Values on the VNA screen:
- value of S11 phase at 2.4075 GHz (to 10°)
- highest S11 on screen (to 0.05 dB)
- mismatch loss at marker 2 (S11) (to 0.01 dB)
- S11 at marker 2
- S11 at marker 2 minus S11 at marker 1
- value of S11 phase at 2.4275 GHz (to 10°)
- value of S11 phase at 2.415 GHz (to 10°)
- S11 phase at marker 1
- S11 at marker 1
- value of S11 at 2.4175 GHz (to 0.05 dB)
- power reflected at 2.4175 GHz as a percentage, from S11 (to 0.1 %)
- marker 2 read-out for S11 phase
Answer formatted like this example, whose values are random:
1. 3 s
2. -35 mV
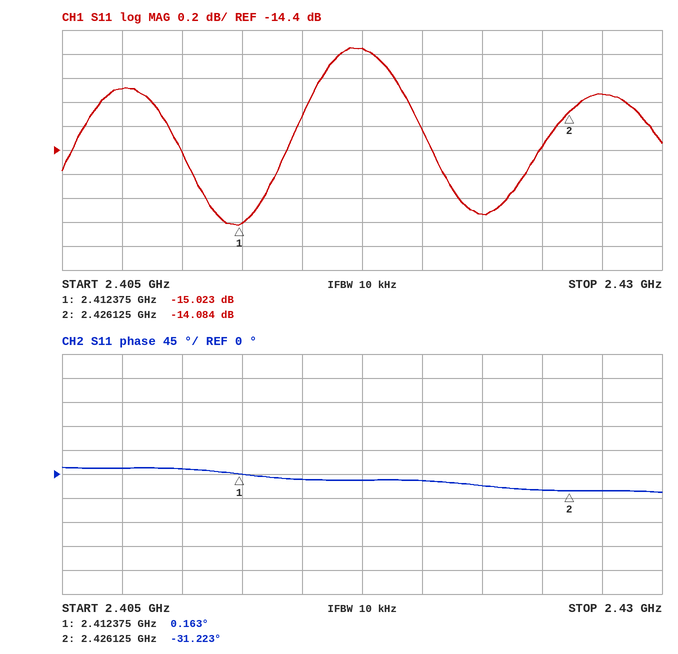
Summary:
1. 10°
2. -13.55 dB
3. 0.17 dB
4. -14.084 dB
5. 0.939 dB
6. -30°
7. -10°
8. 0.163°
9. -15.023 dB
10. -13.55 dB
11. 4.4 %
12. -31.223°
